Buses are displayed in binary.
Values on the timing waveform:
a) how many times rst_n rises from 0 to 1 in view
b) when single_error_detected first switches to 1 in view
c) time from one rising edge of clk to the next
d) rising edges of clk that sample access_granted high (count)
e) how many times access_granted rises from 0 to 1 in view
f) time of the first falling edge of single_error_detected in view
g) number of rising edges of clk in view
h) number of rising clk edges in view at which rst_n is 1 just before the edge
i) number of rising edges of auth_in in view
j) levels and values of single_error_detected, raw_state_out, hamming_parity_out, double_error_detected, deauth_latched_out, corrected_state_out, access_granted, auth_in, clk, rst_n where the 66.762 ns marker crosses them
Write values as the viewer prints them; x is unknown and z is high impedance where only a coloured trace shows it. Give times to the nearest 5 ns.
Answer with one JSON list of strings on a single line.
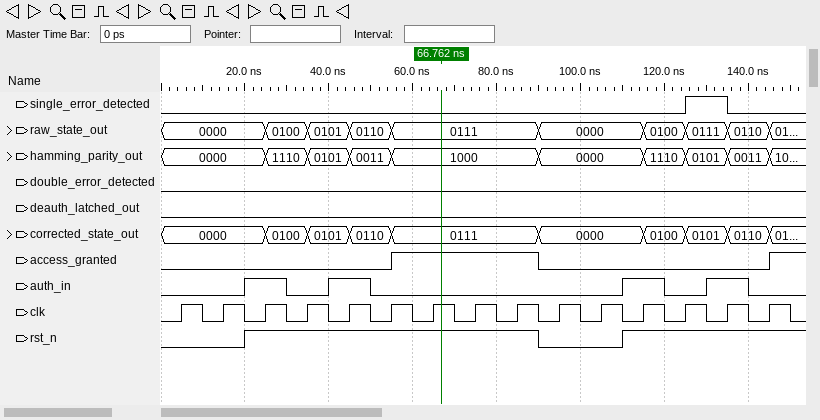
["2", "125 ns", "10 ns", "3", "2", "135 ns", "15", "11", "4", "single_error_detected=0, raw_state_out=0111, hamming_parity_out=1000, double_error_detected=0, deauth_latched_out=0, corrected_state_out=0111, access_granted=1, auth_in=0, clk=1, rst_n=1"]
